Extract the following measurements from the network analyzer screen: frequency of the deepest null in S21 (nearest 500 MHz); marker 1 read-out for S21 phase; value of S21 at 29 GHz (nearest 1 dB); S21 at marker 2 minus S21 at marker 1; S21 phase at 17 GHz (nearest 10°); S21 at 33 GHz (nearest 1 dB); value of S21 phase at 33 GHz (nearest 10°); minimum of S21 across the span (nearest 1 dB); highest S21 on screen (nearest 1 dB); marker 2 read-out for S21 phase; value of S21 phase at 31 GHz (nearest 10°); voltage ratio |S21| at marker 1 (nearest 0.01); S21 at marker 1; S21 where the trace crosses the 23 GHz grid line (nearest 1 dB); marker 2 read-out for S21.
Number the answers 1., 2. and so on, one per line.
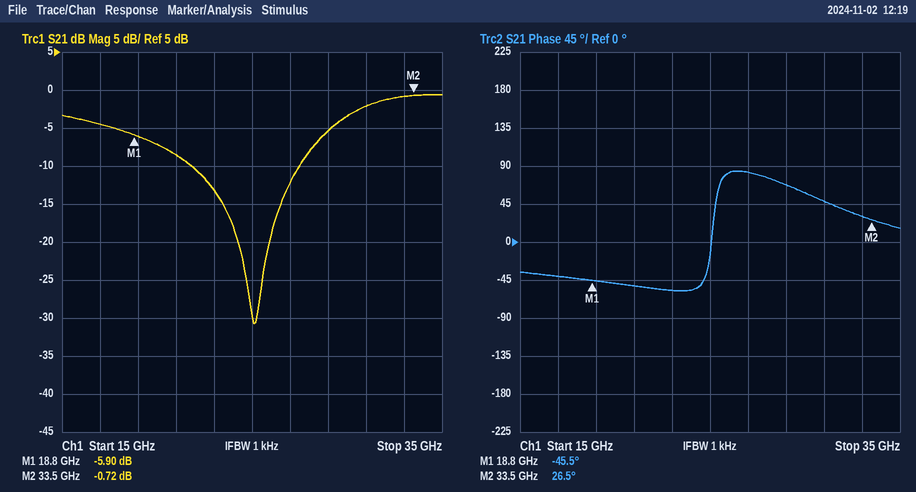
1. 25.0 GHz
2. -45.5°
3. -5 dB
4. 5.18 dB
5. -40°
6. -1 dB
7. 30°
8. -31 dB
9. -1 dB
10. 26.5°
11. 50°
12. 0.51
13. -5.90 dB
14. -13 dB
15. -0.72 dB
